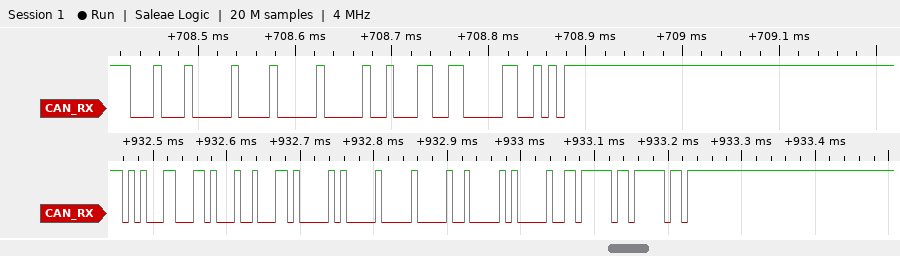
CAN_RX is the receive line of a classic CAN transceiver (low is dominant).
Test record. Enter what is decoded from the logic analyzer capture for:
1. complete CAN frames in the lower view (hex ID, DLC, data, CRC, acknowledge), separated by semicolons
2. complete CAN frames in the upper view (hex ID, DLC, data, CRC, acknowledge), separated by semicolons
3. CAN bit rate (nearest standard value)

ID 14611234, DLC 4, data 00 01 02 03, CRC 3FBF, ACK
ID 110, DLC 2, data 00 11, CRC 4C12, ACK
125 kbit/s
